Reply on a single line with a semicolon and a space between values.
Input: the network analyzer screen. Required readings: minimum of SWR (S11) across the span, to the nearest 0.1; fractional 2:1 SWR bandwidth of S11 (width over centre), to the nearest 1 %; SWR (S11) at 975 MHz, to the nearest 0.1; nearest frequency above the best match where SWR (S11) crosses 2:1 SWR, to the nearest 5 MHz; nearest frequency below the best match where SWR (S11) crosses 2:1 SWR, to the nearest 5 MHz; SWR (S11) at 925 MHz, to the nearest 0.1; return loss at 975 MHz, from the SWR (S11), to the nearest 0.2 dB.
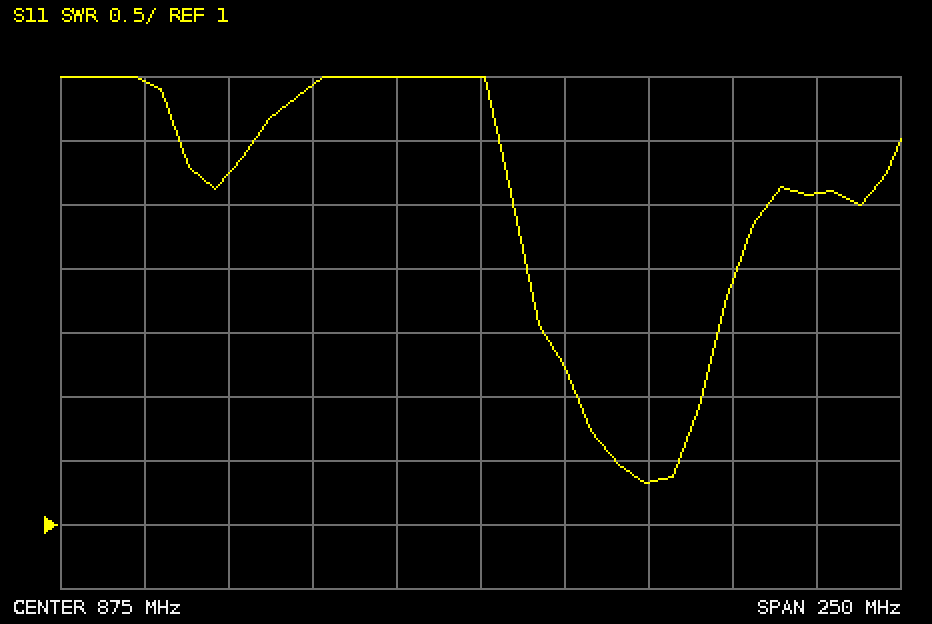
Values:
1.3; 4 %; 3.6; 940 MHz; 905 MHz; 1.3; 5.0 dB
